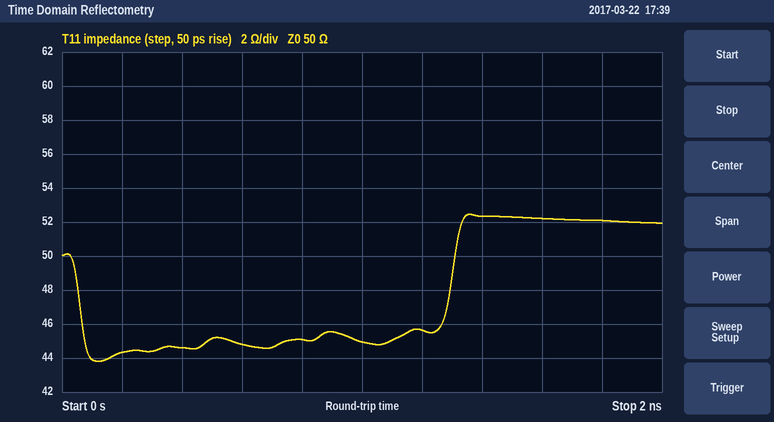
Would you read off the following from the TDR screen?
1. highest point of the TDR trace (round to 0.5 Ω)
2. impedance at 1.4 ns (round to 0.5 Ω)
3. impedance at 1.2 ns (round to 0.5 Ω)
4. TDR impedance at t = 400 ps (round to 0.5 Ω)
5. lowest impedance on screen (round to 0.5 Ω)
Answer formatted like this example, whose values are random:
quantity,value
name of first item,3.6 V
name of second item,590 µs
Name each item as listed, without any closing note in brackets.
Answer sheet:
quantity,value
highest point of the TDR trace,52.5 Ω
impedance at 1.4 ns,52.5 Ω
impedance at 1.2 ns,45.5 Ω
TDR impedance at t = 400 ps,44.5 Ω
lowest impedance on screen,44.0 Ω
